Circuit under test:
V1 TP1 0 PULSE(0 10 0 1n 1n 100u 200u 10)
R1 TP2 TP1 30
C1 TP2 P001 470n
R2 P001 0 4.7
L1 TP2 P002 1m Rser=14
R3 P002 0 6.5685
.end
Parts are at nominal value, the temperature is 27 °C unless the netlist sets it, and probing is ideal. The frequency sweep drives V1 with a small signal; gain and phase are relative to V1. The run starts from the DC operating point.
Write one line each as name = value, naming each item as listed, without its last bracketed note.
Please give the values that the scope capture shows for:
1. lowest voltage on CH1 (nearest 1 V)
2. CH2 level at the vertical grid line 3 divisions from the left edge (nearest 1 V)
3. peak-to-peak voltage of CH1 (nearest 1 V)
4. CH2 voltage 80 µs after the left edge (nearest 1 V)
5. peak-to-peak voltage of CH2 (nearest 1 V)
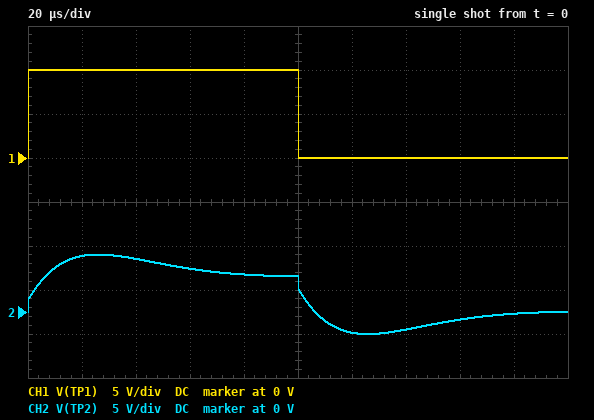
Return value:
lowest voltage on CH1 = 0 V
CH2 level at the vertical grid line 3 divisions from the left edge = 5 V
peak-to-peak voltage of CH1 = 10 V
CH2 voltage 80 µs after the left edge = 4 V
peak-to-peak voltage of CH2 = 9 V
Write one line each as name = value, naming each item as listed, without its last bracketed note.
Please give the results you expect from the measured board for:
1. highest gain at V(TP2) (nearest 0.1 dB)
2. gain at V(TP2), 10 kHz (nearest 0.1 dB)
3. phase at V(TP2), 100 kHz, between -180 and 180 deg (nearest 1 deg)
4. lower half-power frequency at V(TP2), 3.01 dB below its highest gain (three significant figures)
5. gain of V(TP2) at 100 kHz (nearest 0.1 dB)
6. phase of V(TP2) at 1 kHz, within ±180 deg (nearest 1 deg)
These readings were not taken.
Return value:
highest gain at V(TP2) = -2.3 dB
gain at V(TP2), 10 kHz = -2.5 dB
phase at V(TP2), 100 kHz, between -180 and 180 deg = -30 deg
lower half-power frequency at V(TP2), 3.01 dB below its highest gain = 3.10 kHz
gain of V(TP2) at 100 kHz = -15.6 dB
phase of V(TP2) at 1 kHz, within ±180 deg = 8 deg
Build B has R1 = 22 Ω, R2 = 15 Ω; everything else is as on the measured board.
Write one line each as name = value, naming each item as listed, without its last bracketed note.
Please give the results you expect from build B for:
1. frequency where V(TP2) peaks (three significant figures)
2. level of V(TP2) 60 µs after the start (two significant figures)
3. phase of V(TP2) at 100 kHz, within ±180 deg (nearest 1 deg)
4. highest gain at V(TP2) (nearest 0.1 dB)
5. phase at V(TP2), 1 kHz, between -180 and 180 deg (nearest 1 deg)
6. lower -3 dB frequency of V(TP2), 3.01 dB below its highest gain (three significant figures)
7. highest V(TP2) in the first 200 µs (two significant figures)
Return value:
frequency where V(TP2) peaks = 7.52 kHz
level of V(TP2) 60 µs after the start = 5.7 V
phase of V(TP2) at 100 kHz, within ±180 deg = -7 deg
highest gain at V(TP2) = -2.4 dB
phase at V(TP2), 1 kHz, between -180 and 180 deg = 7 deg
lower -3 dB frequency of V(TP2), 3.01 dB below its highest gain = 1.79 kHz
highest V(TP2) in the first 200 µs = 6.8 V
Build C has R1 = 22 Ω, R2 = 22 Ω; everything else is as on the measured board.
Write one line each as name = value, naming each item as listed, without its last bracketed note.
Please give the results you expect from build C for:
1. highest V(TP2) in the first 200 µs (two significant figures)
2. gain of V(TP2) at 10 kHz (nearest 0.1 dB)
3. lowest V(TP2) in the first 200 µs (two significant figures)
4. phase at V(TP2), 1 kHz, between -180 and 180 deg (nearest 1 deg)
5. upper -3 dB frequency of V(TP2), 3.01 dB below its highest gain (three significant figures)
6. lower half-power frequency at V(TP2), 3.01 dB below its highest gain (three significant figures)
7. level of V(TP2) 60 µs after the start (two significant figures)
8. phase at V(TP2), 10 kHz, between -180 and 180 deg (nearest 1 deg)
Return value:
highest V(TP2) in the first 200 µs = 6.6 V
gain of V(TP2) at 10 kHz = -3.0 dB
lowest V(TP2) in the first 200 µs = -1.7 V
phase at V(TP2), 1 kHz, between -180 and 180 deg = 7 deg
upper -3 dB frequency of V(TP2), 3.01 dB below its highest gain = 49.1 kHz
lower half-power frequency at V(TP2), 3.01 dB below its highest gain = 1.45 kHz
level of V(TP2) 60 µs after the start = 5.6 V
phase at V(TP2), 10 kHz, between -180 and 180 deg = -6 deg
